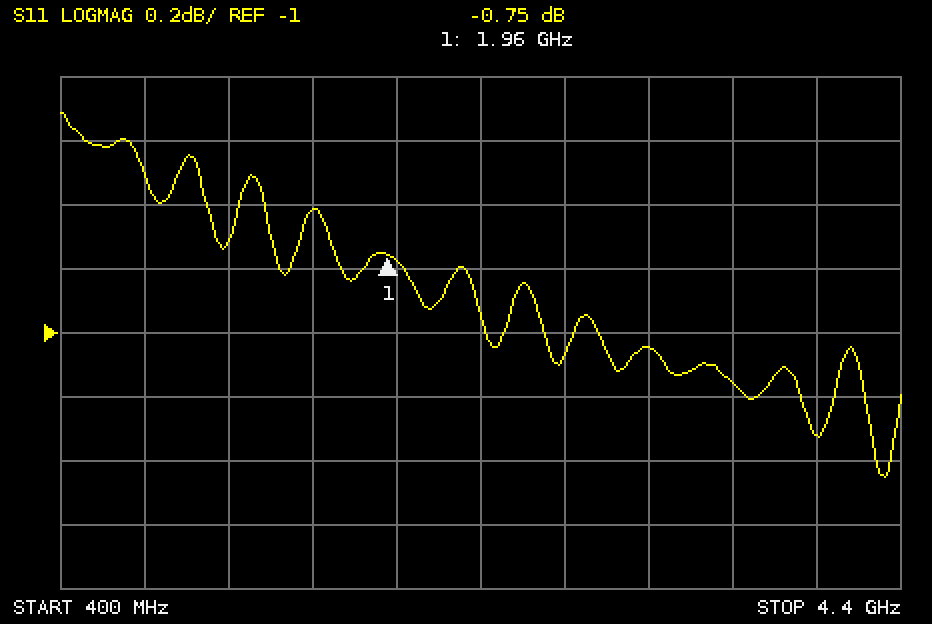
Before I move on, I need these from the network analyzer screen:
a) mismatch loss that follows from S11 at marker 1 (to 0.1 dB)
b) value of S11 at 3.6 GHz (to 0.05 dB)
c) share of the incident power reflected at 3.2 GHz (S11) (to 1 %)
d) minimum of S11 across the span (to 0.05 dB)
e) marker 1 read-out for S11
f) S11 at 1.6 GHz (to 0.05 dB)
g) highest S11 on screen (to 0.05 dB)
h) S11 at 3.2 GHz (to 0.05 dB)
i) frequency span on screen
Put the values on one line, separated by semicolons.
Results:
8.0 dB; -1.15 dB; 79 %; -1.45 dB; -0.75 dB; -0.60 dB; -0.30 dB; -1.05 dB; 4 GHz
